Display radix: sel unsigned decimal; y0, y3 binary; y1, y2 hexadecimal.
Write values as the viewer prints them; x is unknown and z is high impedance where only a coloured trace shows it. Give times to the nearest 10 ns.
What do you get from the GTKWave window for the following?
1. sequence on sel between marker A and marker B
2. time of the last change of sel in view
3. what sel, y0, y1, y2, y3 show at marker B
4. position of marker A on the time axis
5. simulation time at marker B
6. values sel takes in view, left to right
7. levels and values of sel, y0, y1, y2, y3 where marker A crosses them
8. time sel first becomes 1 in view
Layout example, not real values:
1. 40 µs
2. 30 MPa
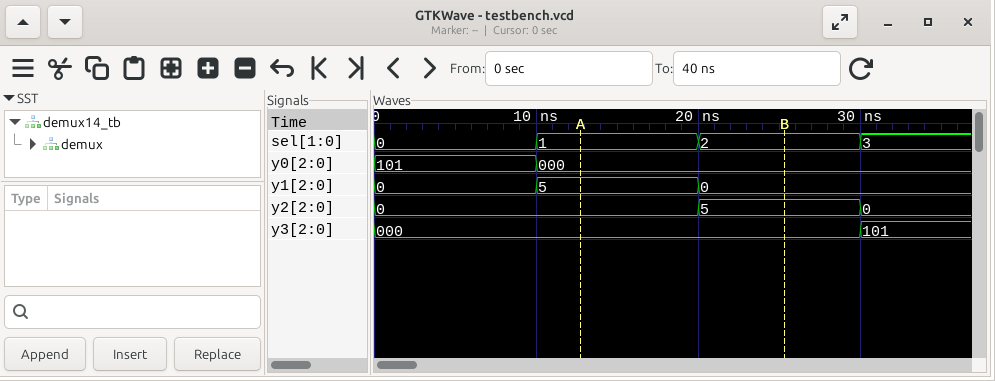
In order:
1. 1, 2
2. 30 ns
3. sel=2, y0=000, y1=0, y2=5, y3=000
4. 10 ns
5. 30 ns
6. 0, 1, 2, 3
7. sel=1, y0=000, y1=5, y2=0, y3=000
8. 10 ns
